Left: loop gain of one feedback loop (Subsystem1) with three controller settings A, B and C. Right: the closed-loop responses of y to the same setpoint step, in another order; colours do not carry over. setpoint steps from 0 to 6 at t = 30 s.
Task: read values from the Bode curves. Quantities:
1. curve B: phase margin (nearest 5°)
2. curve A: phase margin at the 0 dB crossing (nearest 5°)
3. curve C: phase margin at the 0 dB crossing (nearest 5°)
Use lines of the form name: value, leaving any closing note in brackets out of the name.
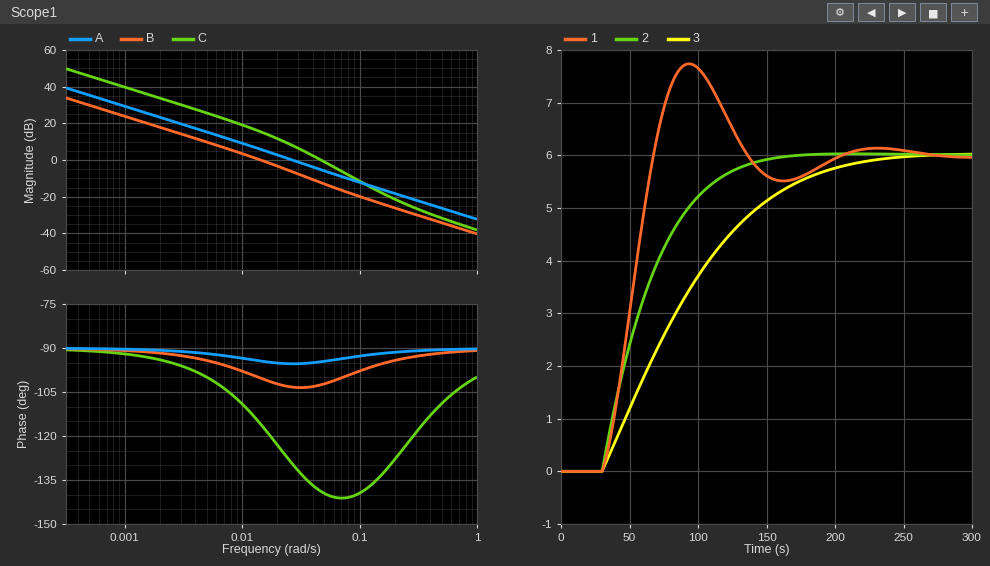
curve B: phase margin: 80°
curve A: phase margin at the 0 dB crossing: 85°
curve C: phase margin at the 0 dB crossing: 40°
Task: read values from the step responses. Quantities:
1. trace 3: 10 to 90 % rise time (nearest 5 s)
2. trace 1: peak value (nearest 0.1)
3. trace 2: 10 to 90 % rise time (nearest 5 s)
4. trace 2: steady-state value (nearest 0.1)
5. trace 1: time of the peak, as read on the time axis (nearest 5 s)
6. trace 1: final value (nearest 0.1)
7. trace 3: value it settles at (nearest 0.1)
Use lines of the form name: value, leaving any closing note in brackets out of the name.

trace 3: 10 to 90 % rise time: 125 s
trace 1: peak value: 7.7
trace 2: 10 to 90 % rise time: 75 s
trace 2: steady-state value: 6.0
trace 1: time of the peak, as read on the time axis: 95 s
trace 1: final value: 6.0
trace 3: value it settles at: 6.0
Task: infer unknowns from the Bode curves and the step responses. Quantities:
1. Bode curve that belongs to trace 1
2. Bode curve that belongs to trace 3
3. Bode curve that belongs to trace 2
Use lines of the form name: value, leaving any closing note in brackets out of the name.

Bode curve that belongs to trace 1: C
Bode curve that belongs to trace 3: B
Bode curve that belongs to trace 2: A
